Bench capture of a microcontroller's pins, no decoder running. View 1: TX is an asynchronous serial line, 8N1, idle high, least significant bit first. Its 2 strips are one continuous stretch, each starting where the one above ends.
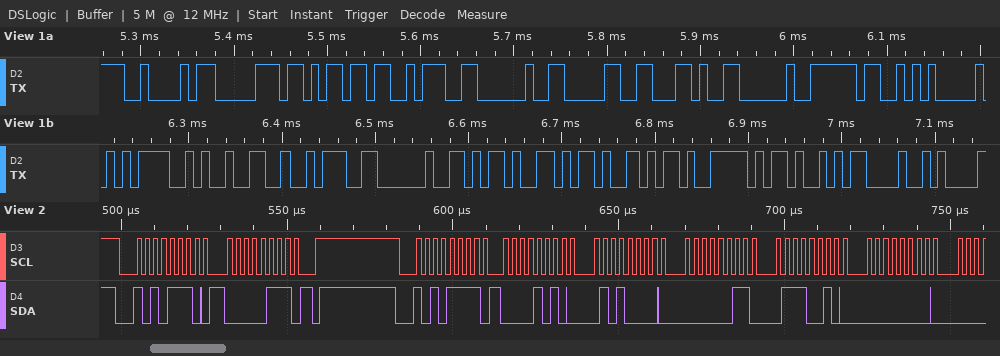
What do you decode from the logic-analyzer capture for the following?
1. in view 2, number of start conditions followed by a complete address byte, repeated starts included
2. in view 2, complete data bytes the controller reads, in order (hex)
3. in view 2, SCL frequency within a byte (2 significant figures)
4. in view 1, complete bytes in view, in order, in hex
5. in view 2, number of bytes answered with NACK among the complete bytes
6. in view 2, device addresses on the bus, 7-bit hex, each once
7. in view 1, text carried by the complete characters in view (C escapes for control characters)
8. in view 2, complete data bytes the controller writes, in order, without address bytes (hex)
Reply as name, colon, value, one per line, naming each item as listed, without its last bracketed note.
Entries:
in view 2, number of start conditions followed by a complete address byte, repeated starts included: 2
in view 2, complete data bytes the controller reads, in order: 0A 50 03 72 00
in view 2, SCL frequency within a byte: 400 kHz
in view 1, complete bytes in view, in order, in hex: 42 70 6D 3A 20 30 2C 20 53 50 4F 32 3A 20 2D 2D 2D 2D 0D 0A
in view 2, number of bytes answered with NACK among the complete bytes: 0
in view 2, device addresses on the bus, 7-bit hex, each once: 0x57
in view 1, text carried by the complete characters in view: "Bpm: 0, SPO2: ----\r\n"
in view 2, complete data bytes the controller writes, in order, without address bytes: 07
